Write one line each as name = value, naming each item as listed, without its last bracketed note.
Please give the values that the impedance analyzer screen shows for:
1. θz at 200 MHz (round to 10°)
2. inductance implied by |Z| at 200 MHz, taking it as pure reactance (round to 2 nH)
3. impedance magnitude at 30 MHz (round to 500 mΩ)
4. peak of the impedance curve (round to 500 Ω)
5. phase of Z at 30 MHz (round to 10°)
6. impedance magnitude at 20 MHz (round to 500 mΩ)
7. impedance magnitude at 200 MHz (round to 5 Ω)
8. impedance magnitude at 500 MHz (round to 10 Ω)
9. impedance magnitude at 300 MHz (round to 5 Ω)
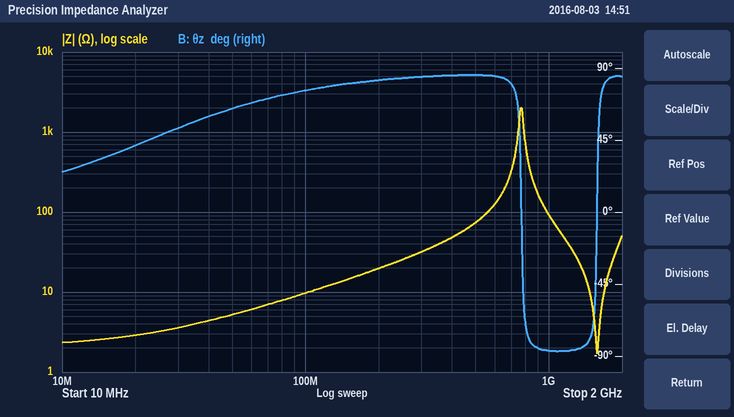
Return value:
θz at 200 MHz = 80°
inductance implied by |Z| at 200 MHz, taking it as pure reactance = 16 nH
impedance magnitude at 30 MHz = 3.5 Ω
peak of the impedance curve = 2.0 kΩ
phase of Z at 30 MHz = 50°
impedance magnitude at 20 MHz = 3.0 Ω
impedance magnitude at 200 MHz = 20 Ω
impedance magnitude at 500 MHz = 70 Ω
impedance magnitude at 300 MHz = 30 Ω
